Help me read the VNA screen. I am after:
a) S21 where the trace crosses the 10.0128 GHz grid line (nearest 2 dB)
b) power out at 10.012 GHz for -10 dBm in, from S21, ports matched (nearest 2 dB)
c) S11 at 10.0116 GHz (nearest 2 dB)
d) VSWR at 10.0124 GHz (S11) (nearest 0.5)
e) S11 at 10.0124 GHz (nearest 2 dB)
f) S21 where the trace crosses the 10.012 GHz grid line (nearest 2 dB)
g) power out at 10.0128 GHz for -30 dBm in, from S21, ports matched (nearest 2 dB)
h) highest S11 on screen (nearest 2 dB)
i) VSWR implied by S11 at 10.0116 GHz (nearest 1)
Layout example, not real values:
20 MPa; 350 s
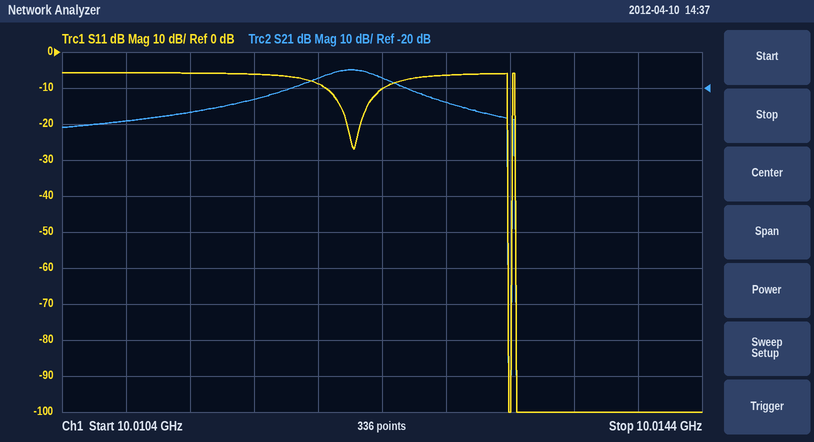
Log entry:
-24 dB; -28 dBm; -6 dB; 2.0; -10 dB; -18 dB; -54 dBm; -6 dB; 3
